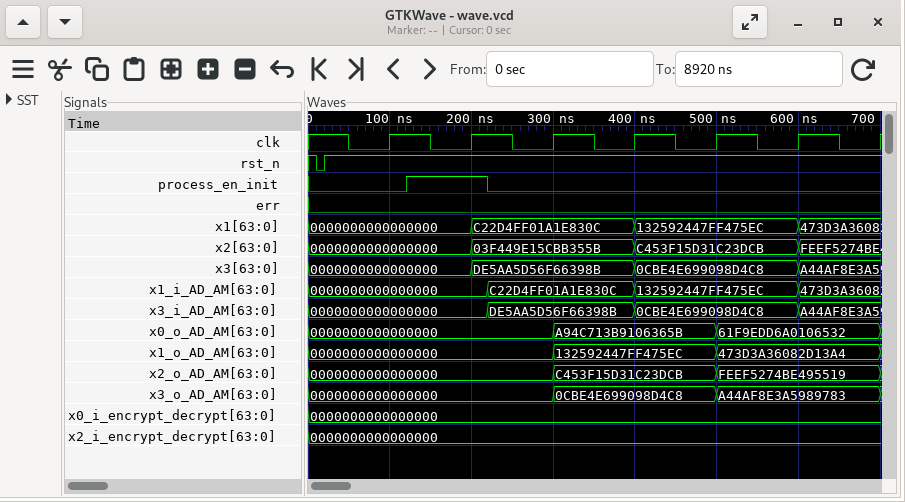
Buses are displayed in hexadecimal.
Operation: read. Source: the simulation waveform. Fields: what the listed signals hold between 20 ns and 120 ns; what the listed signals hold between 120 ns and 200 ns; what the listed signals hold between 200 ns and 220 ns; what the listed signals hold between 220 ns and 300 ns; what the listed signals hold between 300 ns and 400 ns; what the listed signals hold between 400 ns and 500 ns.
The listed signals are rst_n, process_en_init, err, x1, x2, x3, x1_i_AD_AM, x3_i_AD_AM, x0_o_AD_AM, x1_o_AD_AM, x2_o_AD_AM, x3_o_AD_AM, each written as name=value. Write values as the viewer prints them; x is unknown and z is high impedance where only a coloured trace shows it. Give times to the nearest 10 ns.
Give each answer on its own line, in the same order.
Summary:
rst_n=1, process_en_init=0, err=0, x1=0000000000000000, x2=0000000000000000, x3=0000000000000000, x1_i_AD_AM=0000000000000000, x3_i_AD_AM=0000000000000000, x0_o_AD_AM=0000000000000000, x1_o_AD_AM=0000000000000000, x2_o_AD_AM=0000000000000000, x3_o_AD_AM=0000000000000000
rst_n=1, process_en_init=1, err=0, x1=0000000000000000, x2=0000000000000000, x3=0000000000000000, x1_i_AD_AM=0000000000000000, x3_i_AD_AM=0000000000000000, x0_o_AD_AM=0000000000000000, x1_o_AD_AM=0000000000000000, x2_o_AD_AM=0000000000000000, x3_o_AD_AM=0000000000000000
rst_n=1, process_en_init=1, err=0, x1=C22D4FF01A1E830C, x2=03F449E15CBB355B, x3=DE5AA5D56F66398B, x1_i_AD_AM=0000000000000000, x3_i_AD_AM=0000000000000000, x0_o_AD_AM=0000000000000000, x1_o_AD_AM=0000000000000000, x2_o_AD_AM=0000000000000000, x3_o_AD_AM=0000000000000000
rst_n=1, process_en_init=0, err=0, x1=C22D4FF01A1E830C, x2=03F449E15CBB355B, x3=DE5AA5D56F66398B, x1_i_AD_AM=C22D4FF01A1E830C, x3_i_AD_AM=DE5AA5D56F66398B, x0_o_AD_AM=0000000000000000, x1_o_AD_AM=0000000000000000, x2_o_AD_AM=0000000000000000, x3_o_AD_AM=0000000000000000
rst_n=1, process_en_init=0, err=0, x1=C22D4FF01A1E830C, x2=03F449E15CBB355B, x3=DE5AA5D56F66398B, x1_i_AD_AM=C22D4FF01A1E830C, x3_i_AD_AM=DE5AA5D56F66398B, x0_o_AD_AM=A94C713B9106365B, x1_o_AD_AM=132592447FF475EC, x2_o_AD_AM=C453F15D31C23DCB, x3_o_AD_AM=0CBE4E699098D4C8
rst_n=1, process_en_init=0, err=0, x1=132592447FF475EC, x2=C453F15D31C23DCB, x3=0CBE4E699098D4C8, x1_i_AD_AM=132592447FF475EC, x3_i_AD_AM=0CBE4E699098D4C8, x0_o_AD_AM=A94C713B9106365B, x1_o_AD_AM=132592447FF475EC, x2_o_AD_AM=C453F15D31C23DCB, x3_o_AD_AM=0CBE4E699098D4C8
